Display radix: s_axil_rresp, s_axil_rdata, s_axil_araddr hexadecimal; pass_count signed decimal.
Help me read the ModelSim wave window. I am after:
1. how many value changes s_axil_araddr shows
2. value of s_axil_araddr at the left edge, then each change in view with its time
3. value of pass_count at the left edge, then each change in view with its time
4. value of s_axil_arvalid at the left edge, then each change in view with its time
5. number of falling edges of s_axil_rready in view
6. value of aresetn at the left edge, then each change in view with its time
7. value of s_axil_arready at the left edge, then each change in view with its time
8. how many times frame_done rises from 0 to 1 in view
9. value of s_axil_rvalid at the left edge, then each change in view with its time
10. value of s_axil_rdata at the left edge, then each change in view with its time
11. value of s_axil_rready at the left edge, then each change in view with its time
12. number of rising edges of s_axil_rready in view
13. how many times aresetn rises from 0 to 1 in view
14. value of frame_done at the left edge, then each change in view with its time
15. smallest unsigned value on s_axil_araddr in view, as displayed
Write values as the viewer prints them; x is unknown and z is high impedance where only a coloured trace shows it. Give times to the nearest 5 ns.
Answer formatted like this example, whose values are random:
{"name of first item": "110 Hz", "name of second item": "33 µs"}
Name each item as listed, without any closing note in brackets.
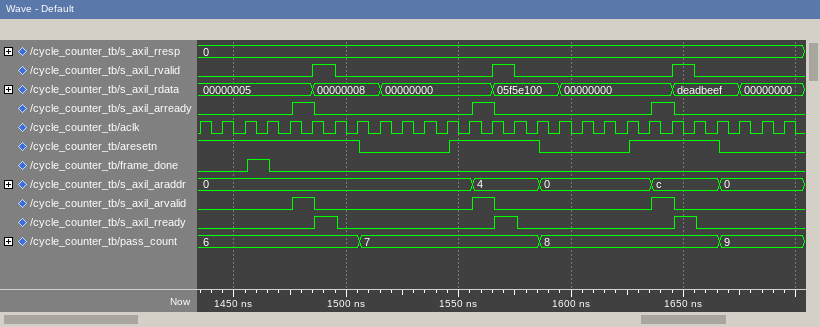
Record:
{"how many value changes s_axil_araddr shows": "4", "value of s_axil_araddr at the left edge, then each change in view with its time": "0, 4 at 1555 ns, 0 at 1585 ns, c at 1635 ns, 0 at 1665 ns", "value of pass_count at the left edge, then each change in view with its time": "6, 7 at 1505 ns, 8 at 1585 ns, 9 at 1665 ns", "value of s_axil_arvalid at the left edge, then each change in view with its time": "0, 1 at 1475 ns, 0 at 1485 ns, 1 at 1555 ns, 0 at 1565 ns, 1 at 1635 ns, 0 at 1645 ns", "number of falling edges of s_axil_rready in view": "3", "value of aresetn at the left edge, then each change in view with its time": "1, 0 at 1505 ns, 1 at 1545 ns, 0 at 1585 ns, 1 at 1625 ns, 0 at 1665 ns", "value of s_axil_arready at the left edge, then each change in view with its time": "0, 1 at 1475 ns, 0 at 1485 ns, 1 at 1555 ns, 0 at 1565 ns, 1 at 1635 ns, 0 at 1645 ns", "how many times frame_done rises from 0 to 1 in view": "1", "value of s_axil_rvalid at the left edge, then each change in view with its time": "0, 1 at 1485 ns, 0 at 1495 ns, 1 at 1565 ns, 0 at 1575 ns, 1 at 1645 ns, 0 at 1655 ns", "value of s_axil_rdata at the left edge, then each change in view with its time": "00000005, 00000008 at 1485 ns, 00000000 at 1515 ns, 05f5e100 at 1565 ns, 00000000 at 1595 ns, deadbeef at 1645 ns, 00000000 at 1675 ns", "value of s_axil_rready at the left edge, then each change in view with its time": "0, 1 at 1485 ns, 0 at 1495 ns, 1 at 1565 ns, 0 at 1575 ns, 1 at 1645 ns, 0 at 1655 ns", "number of rising edges of s_axil_rready in view": "3", "how many times aresetn rises from 0 to 1 in view": "2", "value of frame_done at the left edge, then each change in view with its time": "0, 1 at 1455 ns, 0 at 1465 ns", "smallest unsigned value on s_axil_araddr in view, as displayed": "0"}
